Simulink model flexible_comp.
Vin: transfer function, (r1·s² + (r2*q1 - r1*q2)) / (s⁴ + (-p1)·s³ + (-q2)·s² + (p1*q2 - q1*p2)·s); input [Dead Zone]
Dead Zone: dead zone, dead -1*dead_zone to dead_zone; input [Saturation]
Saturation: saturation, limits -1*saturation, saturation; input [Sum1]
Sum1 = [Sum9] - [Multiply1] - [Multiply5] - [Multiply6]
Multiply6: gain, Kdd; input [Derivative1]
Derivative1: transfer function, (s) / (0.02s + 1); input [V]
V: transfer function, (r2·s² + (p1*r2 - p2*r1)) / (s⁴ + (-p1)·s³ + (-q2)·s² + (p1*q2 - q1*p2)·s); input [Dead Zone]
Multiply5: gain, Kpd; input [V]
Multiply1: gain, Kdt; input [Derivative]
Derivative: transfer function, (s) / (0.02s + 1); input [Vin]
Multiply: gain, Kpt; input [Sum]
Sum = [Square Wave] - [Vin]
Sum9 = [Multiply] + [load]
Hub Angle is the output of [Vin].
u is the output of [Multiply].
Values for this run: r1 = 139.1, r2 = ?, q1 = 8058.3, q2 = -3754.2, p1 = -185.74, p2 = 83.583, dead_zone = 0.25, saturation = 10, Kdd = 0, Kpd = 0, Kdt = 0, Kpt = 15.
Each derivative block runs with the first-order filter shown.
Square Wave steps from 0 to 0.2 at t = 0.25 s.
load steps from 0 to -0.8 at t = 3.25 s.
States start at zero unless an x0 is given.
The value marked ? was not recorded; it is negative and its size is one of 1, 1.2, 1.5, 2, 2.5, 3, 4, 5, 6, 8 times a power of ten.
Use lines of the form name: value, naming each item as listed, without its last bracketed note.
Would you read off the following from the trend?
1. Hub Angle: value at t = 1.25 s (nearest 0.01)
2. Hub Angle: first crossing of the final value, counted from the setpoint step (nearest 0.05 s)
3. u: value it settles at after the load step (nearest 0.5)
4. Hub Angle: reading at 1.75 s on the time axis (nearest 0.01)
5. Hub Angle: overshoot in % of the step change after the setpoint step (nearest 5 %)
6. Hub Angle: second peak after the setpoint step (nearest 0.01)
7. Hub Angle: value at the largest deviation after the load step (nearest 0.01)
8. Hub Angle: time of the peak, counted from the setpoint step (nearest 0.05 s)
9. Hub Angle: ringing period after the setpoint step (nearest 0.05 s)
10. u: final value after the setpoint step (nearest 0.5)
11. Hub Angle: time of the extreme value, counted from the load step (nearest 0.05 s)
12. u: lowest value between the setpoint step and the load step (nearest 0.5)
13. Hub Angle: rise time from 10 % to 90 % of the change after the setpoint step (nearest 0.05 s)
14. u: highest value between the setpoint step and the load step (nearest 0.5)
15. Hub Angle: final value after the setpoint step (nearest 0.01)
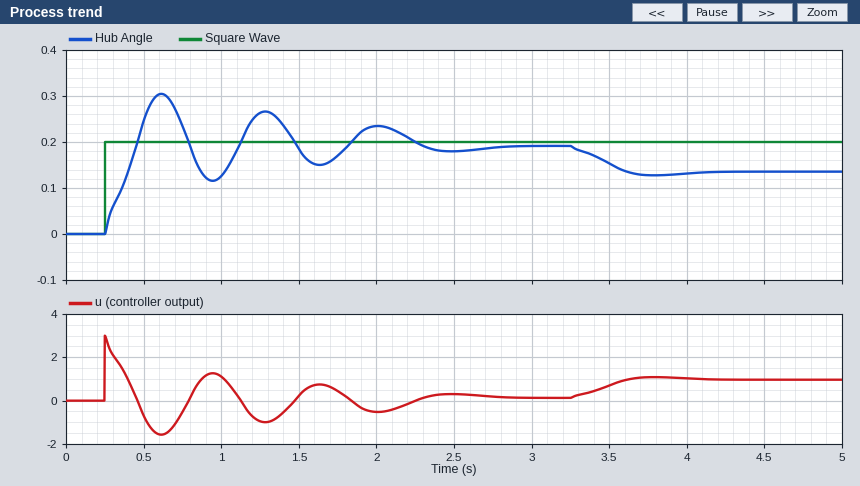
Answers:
Hub Angle: value at t = 1.25 s: 0.26
Hub Angle: first crossing of the final value, counted from the setpoint step: 0.20 s
u: value it settles at after the load step: 1.0
Hub Angle: reading at 1.75 s on the time axis: 0.17
Hub Angle: overshoot in % of the step change after the setpoint step: 60 %
Hub Angle: second peak after the setpoint step: 0.27
Hub Angle: value at the largest deviation after the load step: 0.13
Hub Angle: time of the peak, counted from the setpoint step: 0.35 s
Hub Angle: ringing period after the setpoint step: 0.65 s
u: final value after the setpoint step: 0.0
Hub Angle: time of the extreme value, counted from the load step: 0.55 s
u: lowest value between the setpoint step and the load step: -1.5
Hub Angle: rise time from 10 % to 90 % of the change after the setpoint step: 0.15 s
u: highest value between the setpoint step and the load step: 3.0
Hub Angle: final value after the setpoint step: 0.19
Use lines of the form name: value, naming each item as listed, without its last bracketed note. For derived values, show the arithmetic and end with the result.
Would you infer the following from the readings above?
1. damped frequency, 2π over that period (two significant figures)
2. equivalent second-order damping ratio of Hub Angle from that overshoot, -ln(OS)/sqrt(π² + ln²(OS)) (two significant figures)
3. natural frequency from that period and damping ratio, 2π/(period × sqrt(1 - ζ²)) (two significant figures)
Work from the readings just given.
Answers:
damped frequency, 2π over that period: 2π / 0.65 = 9.7 rad/s
equivalent second-order damping ratio of Hub Angle from that overshoot, -ln(OS)/sqrt(π² + ln²(OS)): ln(0.6) = -0.511; 0.511 / sqrt(9.870 + 0.261) = 0.16
natural frequency from that period and damping ratio, 2π/(period × sqrt(1 - ζ²)): 2π / (0.65 × sqrt(1 - 0.16²)) = 9.8 rad/s
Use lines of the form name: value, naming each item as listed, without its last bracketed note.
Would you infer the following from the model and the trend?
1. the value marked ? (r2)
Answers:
the value marked ?: -60
